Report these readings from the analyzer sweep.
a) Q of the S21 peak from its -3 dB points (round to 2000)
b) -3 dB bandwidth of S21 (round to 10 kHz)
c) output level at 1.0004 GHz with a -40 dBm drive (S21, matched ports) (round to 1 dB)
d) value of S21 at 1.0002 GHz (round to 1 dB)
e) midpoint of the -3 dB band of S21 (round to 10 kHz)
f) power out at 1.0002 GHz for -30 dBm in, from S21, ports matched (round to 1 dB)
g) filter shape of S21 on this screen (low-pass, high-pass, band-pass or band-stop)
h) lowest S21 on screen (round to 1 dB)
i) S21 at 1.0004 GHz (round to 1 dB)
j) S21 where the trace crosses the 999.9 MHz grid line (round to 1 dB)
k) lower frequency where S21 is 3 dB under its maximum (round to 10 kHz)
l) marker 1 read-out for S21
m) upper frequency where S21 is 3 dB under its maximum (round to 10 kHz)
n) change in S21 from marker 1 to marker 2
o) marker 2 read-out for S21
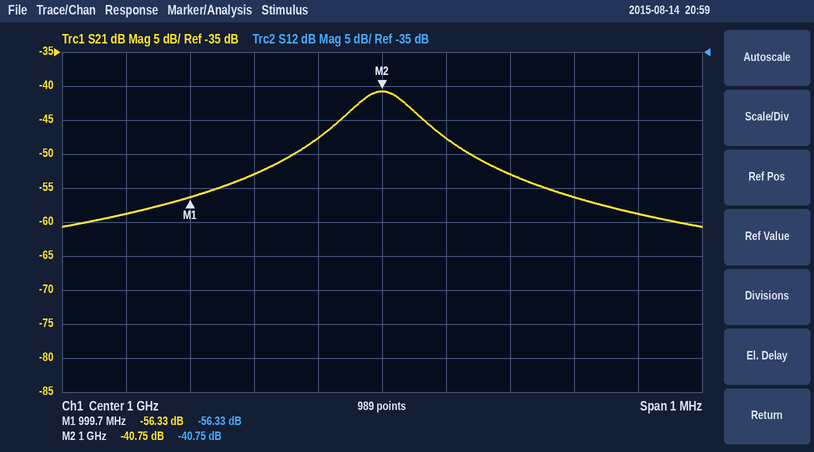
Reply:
10000
100 kHz
-99 dBm
-53 dB
1.00000 GHz
-83 dBm
band-pass
-61 dB
-59 dB
-48 dB
999.95 MHz
-56.33 dB
1.00005 GHz
15.58 dB
-40.75 dB
